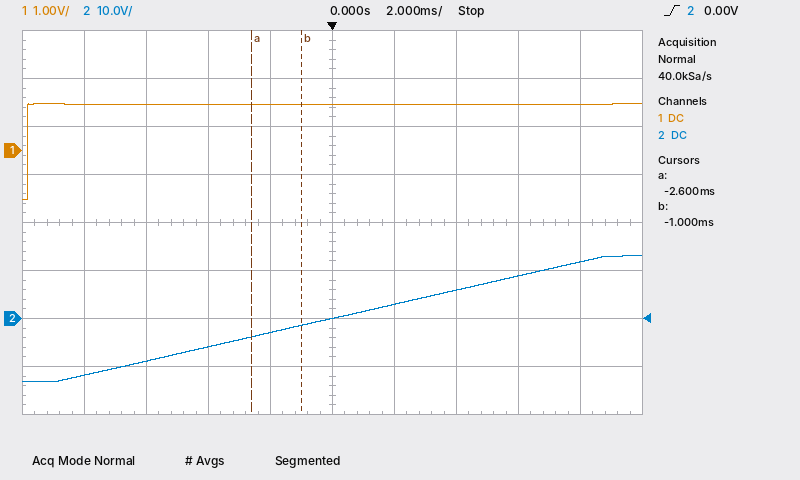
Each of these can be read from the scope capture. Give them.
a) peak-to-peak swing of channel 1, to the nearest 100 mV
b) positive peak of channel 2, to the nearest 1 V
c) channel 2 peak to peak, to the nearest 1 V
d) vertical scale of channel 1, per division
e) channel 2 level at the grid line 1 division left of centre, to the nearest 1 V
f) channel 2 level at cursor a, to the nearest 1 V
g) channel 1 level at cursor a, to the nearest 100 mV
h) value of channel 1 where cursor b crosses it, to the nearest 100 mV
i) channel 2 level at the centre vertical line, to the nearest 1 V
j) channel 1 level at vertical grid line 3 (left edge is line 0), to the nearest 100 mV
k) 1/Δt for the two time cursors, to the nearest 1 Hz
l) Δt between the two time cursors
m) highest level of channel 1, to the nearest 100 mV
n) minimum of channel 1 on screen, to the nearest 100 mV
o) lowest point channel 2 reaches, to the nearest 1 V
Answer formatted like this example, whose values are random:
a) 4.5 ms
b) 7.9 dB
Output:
a) 2.0 V
b) 13 V
c) 26 V
d) 1 V
e) -3 V
f) -4 V
g) 1.0 V
h) 1.0 V
i) 0 V
j) 1.0 V
k) 625 Hz
l) 1.6 ms
m) 1.0 V
n) -1.0 V
o) -13 V
